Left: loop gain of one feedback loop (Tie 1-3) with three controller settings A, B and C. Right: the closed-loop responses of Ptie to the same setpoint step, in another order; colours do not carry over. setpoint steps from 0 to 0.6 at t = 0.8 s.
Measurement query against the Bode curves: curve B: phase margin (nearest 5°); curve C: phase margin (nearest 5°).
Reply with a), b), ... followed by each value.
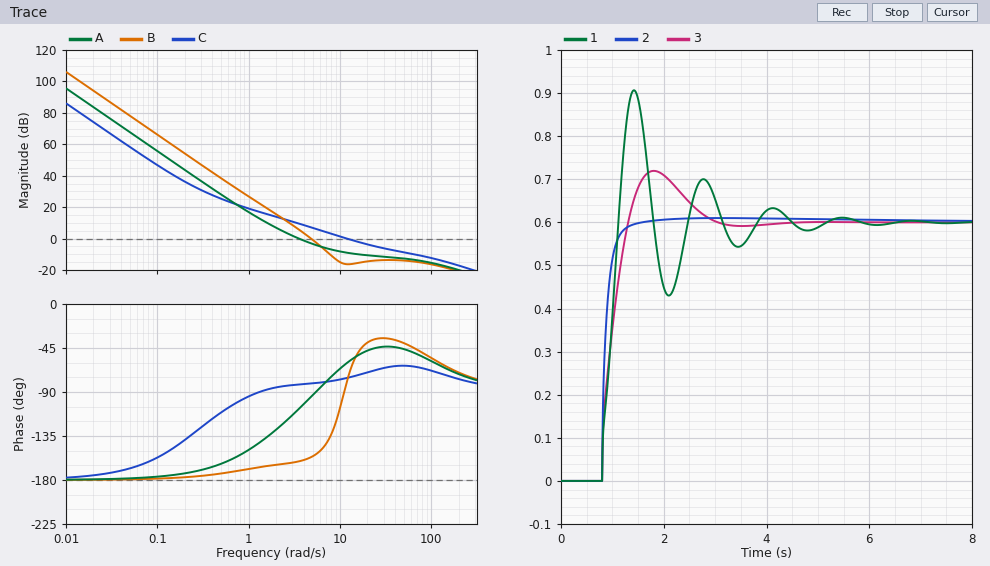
a) 25°
b) 105°
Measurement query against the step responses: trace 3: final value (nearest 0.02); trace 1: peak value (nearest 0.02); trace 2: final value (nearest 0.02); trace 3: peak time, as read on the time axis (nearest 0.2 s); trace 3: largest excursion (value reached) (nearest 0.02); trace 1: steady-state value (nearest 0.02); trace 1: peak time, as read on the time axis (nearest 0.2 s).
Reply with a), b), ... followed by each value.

a) 0.60
b) 0.90
c) 0.60
d) 1.8 s
e) 0.72
f) 0.60
g) 1.4 s
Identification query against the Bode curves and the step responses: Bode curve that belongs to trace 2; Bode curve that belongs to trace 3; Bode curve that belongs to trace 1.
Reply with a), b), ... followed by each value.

a) C
b) A
c) B
